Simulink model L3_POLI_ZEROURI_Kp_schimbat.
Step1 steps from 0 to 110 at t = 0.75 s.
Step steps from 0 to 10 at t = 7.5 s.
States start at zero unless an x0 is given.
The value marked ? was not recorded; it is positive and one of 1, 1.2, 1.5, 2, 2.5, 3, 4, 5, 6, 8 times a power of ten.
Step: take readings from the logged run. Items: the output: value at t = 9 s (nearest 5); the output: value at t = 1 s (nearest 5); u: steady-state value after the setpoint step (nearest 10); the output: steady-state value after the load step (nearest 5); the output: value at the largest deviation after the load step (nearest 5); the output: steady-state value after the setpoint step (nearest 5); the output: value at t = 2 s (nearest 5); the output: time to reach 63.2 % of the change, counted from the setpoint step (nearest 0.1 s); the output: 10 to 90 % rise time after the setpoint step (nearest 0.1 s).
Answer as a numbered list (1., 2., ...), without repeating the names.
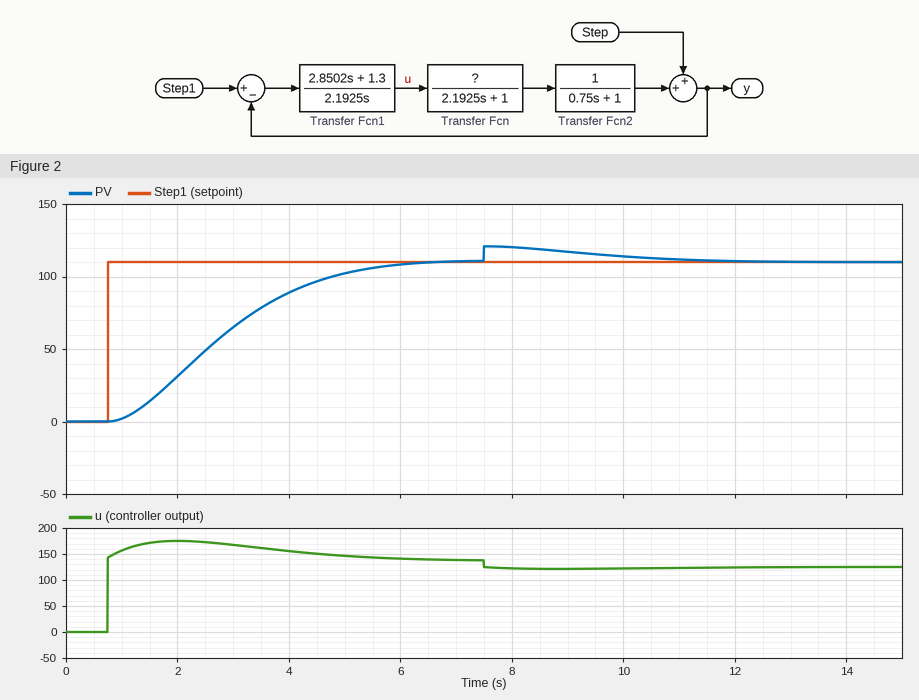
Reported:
1. 115
2. 0
3. 140
4. 110
5. 120
6. 110
7. 30
8. 2.4 s
9. 3.3 s
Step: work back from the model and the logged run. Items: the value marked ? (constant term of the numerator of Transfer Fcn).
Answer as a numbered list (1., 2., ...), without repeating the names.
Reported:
1. 0.8
